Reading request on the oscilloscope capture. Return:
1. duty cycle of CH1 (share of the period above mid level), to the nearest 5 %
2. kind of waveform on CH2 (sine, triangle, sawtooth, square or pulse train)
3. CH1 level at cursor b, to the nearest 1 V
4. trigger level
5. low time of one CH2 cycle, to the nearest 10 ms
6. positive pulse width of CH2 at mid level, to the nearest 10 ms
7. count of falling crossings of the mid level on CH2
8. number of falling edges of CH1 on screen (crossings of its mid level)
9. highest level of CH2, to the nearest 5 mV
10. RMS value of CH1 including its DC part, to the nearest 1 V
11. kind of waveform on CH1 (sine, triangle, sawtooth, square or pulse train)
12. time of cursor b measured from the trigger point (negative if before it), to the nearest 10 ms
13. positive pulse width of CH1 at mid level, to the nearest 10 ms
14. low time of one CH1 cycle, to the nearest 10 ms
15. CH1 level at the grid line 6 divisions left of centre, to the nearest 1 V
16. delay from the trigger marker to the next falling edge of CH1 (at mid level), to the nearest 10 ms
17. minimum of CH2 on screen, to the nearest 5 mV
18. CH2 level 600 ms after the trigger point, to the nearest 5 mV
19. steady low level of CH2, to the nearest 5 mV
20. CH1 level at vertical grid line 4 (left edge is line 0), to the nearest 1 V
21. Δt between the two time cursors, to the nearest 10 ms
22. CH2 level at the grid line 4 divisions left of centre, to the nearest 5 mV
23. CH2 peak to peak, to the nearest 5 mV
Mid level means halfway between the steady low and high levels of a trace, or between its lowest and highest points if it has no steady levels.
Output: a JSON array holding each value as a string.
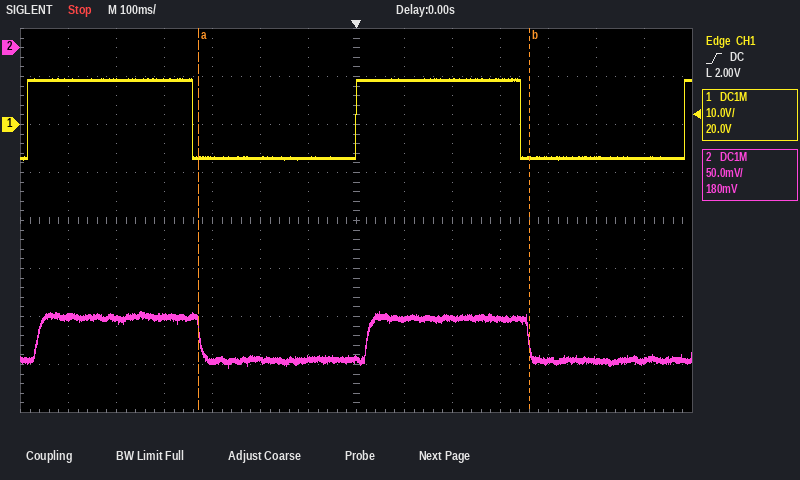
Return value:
["50 %", "square", "-7 V", "2.00 V", "350 ms", "340 ms", "2", "2", "-275 mV", "8 V", "square", "+360 ms", "340 ms", "340 ms", "9 V", "340 ms", "-335 mV", "-325 mV", "-325 mV", "-7 V", "690 ms", "-280 mV", "60 mV"]
